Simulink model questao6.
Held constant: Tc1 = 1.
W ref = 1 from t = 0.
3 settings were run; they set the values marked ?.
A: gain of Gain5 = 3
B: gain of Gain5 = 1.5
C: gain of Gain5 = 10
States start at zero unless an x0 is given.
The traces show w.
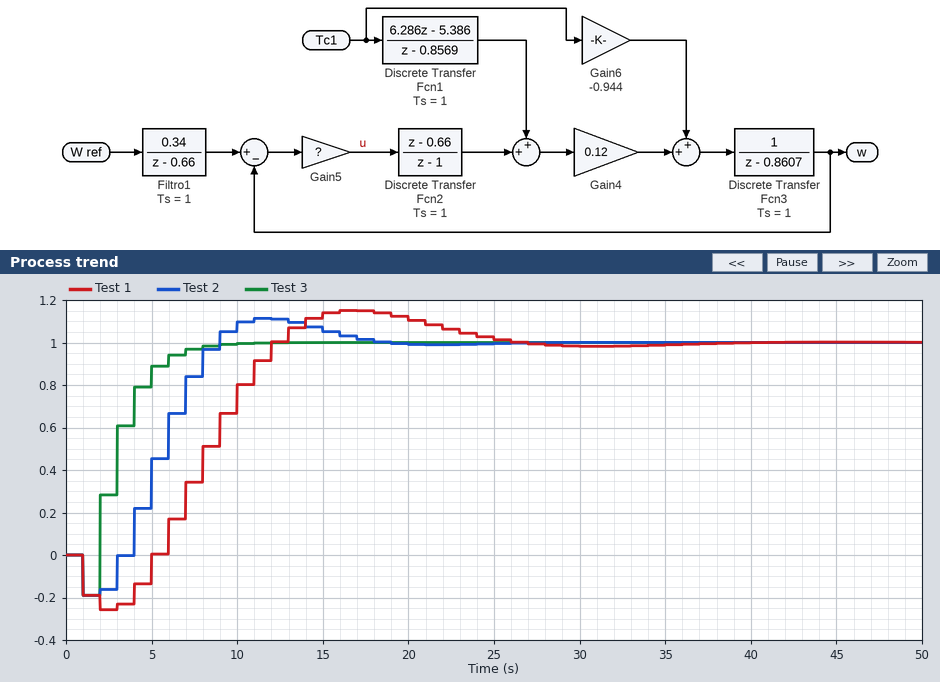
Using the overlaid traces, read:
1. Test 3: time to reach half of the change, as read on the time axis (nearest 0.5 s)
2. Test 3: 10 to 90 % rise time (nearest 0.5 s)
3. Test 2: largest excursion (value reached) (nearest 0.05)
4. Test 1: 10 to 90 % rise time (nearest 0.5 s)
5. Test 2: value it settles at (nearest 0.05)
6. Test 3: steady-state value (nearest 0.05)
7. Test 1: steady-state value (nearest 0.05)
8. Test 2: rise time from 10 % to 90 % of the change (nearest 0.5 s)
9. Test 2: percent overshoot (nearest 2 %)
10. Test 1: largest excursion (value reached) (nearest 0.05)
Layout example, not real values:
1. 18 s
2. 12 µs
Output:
1. 3.0 s
2. 4.0 s
3. 1.10
4. 5.0 s
5. 1.00
6. 1.00
7. 1.00
8. 4.0 s
9. 12 %
10. 1.15
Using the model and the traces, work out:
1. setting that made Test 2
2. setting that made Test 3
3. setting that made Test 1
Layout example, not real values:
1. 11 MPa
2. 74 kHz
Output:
1. A
2. C
3. B
